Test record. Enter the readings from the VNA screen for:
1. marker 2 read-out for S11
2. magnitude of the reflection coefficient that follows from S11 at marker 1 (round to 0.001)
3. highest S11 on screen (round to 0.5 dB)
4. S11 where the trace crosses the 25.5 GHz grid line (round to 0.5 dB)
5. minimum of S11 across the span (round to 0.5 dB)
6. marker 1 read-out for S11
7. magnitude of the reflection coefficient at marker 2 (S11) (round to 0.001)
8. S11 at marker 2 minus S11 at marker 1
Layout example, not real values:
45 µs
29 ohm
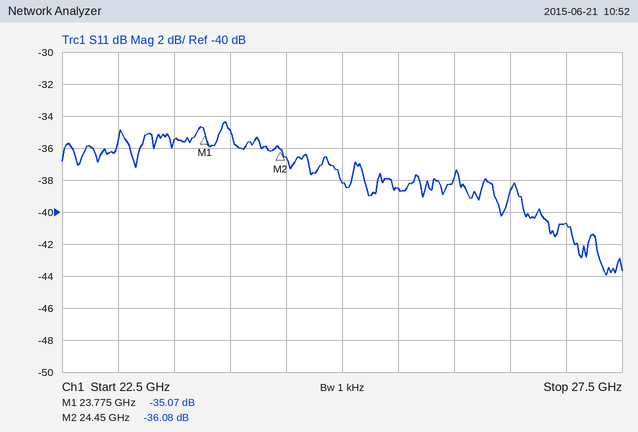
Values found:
-36.08 dB
0.018
-34.5 dB
-38.5 dB
-44.0 dB
-35.07 dB
0.016
-1.01 dB
